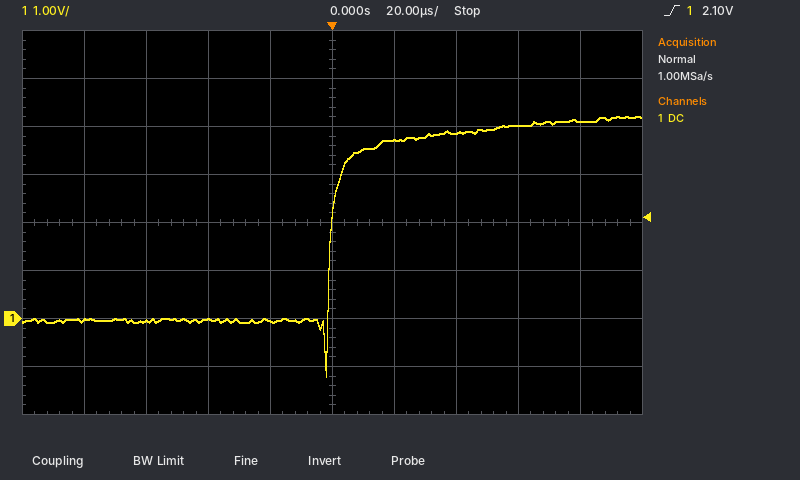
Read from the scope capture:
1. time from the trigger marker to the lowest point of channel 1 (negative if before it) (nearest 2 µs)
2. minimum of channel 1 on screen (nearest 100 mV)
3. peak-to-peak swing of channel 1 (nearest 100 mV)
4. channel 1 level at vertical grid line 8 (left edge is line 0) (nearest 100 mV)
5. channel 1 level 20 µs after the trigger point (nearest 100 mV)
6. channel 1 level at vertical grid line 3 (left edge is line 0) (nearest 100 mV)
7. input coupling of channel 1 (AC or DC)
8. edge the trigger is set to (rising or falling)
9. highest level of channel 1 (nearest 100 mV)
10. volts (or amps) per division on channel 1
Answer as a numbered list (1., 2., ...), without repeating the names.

1. -2 µs
2. -1.2 V
3. 5.4 V
4. 4.0 V
5. 3.7 V
6. 0.0 V
7. DC
8. rising
9. 4.2 V
10. 1 V
